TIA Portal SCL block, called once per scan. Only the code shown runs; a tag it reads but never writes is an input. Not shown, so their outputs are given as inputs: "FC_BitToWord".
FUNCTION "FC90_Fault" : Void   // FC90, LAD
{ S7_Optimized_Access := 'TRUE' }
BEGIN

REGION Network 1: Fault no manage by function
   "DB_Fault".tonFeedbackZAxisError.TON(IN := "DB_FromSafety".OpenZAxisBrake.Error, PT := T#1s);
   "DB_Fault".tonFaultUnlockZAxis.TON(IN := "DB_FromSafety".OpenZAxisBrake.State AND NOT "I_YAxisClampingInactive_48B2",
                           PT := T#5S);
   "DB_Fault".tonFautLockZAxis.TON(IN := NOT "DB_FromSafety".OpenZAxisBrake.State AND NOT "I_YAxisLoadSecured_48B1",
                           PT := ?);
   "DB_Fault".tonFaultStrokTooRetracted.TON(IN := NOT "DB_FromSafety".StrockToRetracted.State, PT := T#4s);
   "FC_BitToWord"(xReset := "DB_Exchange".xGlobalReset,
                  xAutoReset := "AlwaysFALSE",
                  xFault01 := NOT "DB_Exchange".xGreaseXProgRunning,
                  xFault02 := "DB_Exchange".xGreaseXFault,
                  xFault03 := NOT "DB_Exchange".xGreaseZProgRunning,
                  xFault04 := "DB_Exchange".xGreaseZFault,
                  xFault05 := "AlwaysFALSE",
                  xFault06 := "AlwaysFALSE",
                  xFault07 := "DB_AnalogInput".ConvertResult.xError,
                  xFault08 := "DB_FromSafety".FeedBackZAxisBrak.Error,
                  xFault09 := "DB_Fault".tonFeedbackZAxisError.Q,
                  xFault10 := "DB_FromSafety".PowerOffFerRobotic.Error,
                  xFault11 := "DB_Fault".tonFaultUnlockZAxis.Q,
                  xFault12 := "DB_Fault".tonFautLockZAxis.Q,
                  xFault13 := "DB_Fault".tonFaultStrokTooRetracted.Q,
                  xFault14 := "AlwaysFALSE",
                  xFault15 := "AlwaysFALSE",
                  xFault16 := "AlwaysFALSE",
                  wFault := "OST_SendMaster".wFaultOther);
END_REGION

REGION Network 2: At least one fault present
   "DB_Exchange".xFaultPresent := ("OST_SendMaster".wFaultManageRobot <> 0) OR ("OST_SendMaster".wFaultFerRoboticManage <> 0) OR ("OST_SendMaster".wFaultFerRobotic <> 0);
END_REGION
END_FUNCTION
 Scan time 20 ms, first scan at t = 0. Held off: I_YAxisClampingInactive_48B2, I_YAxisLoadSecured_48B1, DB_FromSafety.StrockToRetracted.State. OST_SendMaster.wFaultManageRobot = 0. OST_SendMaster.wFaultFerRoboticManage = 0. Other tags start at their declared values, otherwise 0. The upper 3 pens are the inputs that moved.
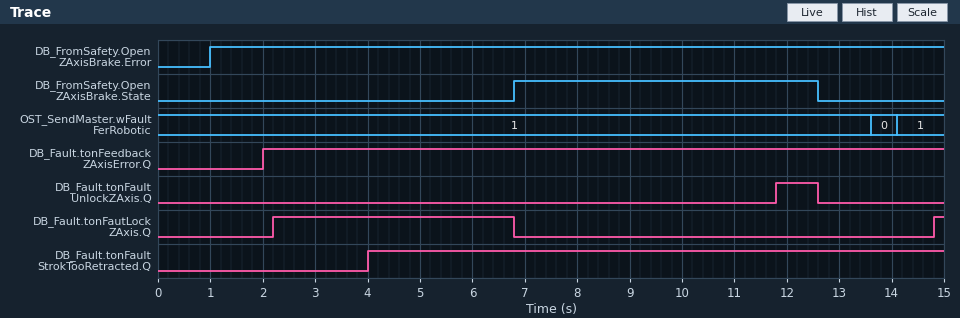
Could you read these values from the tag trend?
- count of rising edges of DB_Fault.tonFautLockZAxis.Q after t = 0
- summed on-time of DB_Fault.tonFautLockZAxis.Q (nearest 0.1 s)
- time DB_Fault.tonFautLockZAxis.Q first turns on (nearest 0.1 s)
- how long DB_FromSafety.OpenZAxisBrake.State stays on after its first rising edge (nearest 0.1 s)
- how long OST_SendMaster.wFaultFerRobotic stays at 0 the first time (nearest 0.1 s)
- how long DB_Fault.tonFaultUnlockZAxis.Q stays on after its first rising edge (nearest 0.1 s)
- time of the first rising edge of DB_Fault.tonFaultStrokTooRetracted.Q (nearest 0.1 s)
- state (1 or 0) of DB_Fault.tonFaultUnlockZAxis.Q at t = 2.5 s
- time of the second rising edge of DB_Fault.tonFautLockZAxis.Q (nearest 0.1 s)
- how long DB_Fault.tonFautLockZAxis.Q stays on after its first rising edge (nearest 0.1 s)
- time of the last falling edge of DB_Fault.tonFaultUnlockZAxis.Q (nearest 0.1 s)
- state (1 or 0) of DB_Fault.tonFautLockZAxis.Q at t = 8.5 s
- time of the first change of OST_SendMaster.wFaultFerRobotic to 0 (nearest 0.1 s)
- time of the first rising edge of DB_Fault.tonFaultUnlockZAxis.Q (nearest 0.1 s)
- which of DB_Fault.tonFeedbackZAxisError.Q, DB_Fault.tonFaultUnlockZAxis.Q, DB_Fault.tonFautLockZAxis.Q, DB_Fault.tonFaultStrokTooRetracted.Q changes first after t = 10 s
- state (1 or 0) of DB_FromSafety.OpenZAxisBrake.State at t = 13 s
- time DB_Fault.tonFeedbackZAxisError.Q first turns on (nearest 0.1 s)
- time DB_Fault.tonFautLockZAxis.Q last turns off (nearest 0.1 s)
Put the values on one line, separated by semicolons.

2; 4.8 s; 2.2 s; 5.8 s; 0.5 s; 0.8 s; 4.0 s; 0; 14.8 s; 4.6 s; 12.6 s; 0; 13.6 s; 11.8 s; DB_Fault.tonFaultUnlockZAxis.Q; 0; 2.0 s; 6.8 s
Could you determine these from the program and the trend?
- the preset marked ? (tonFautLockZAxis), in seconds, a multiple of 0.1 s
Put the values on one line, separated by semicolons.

2.2 s
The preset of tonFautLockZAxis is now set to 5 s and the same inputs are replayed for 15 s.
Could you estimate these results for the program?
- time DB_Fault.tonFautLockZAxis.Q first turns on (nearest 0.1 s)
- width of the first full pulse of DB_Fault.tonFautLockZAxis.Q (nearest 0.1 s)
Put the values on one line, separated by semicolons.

5.0 s; 1.8 s
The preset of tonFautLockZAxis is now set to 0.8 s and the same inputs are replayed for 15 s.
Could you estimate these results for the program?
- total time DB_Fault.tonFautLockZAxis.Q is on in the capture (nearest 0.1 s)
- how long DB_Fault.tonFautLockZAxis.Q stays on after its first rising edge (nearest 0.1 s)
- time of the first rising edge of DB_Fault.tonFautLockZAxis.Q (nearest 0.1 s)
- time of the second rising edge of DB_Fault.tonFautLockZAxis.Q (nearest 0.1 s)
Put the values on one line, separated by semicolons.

7.6 s; 6.0 s; 0.8 s; 13.4 s
